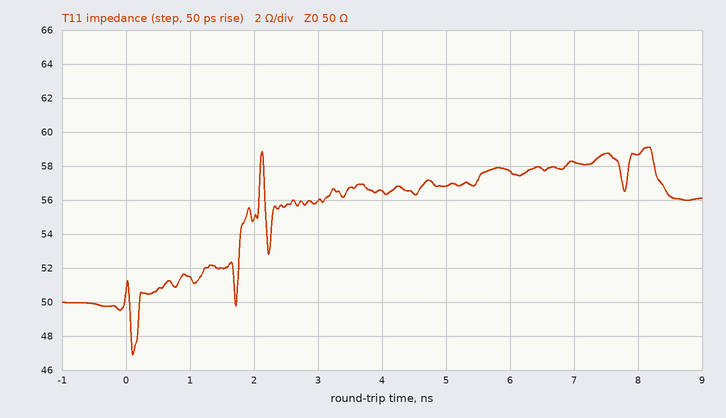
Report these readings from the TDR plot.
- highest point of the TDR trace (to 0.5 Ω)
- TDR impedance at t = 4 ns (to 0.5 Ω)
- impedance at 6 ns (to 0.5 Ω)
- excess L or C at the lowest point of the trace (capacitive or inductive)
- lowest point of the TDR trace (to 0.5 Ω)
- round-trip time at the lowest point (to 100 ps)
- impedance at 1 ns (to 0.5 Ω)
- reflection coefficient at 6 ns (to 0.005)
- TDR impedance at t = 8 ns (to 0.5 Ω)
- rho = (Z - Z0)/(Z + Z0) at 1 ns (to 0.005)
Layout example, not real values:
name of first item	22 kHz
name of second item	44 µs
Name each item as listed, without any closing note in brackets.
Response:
highest point of the TDR trace	59.0 Ω
TDR impedance at t = 4 ns	56.5 Ω
impedance at 6 ns	57.5 Ω
excess L or C at the lowest point of the trace	capacitive
lowest point of the TDR trace	47.0 Ω
round-trip time at the lowest point	100 ps
impedance at 1 ns	51.5 Ω
reflection coefficient at 6 ns	+0.070
TDR impedance at t = 8 ns	58.5 Ω
rho = (Z - Z0)/(Z + Z0) at 1 ns	+0.015
